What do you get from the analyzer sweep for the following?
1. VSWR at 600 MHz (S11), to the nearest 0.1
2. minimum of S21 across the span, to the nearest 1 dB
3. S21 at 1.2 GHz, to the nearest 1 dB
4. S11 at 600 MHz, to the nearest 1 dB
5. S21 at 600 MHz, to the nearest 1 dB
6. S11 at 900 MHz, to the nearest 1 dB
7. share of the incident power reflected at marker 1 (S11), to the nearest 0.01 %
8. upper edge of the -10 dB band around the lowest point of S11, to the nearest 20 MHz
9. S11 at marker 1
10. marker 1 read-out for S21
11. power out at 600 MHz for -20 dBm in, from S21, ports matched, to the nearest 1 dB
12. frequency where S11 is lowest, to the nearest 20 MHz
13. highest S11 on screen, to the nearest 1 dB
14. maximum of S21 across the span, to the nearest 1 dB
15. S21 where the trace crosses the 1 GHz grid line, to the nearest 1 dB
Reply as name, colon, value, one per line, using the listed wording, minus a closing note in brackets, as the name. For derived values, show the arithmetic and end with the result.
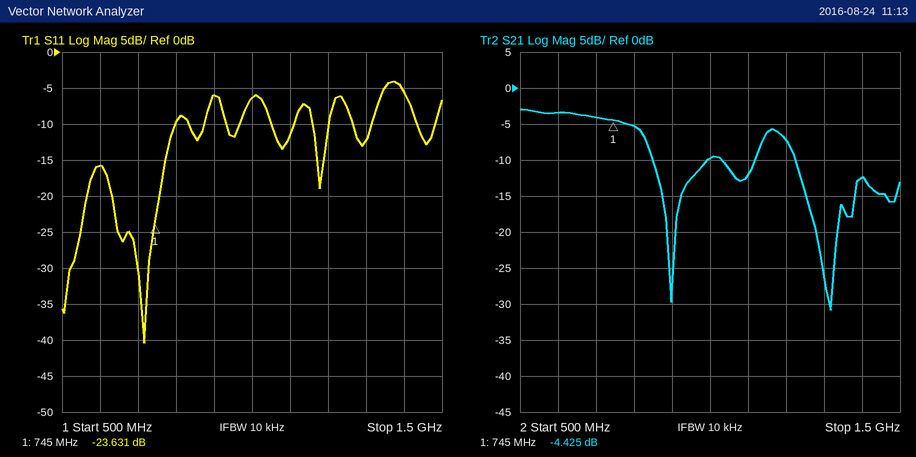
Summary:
VSWR at 600 MHz (S11), to the nearest 0.1: |Γ| = 10^(-16/20) = 0.1585; VSWR = (1 + 0.1585)/(1 − 0.1585) ≈ 1.4
minimum of S21 across the span, to the nearest 1 dB: -31 dB
S21 at 1.2 GHz, to the nearest 1 dB: -7 dB
S11 at 600 MHz, to the nearest 1 dB: -16 dB
S21 at 600 MHz, to the nearest 1 dB: -3 dB
S11 at 900 MHz, to the nearest 1 dB: -6 dB
share of the incident power reflected at marker 1 (S11), to the nearest 0.01 %: 10^(-23.631/10) ≈ 0.43 %
upper edge of the -10 dB band around the lowest point of S11, to the nearest 20 MHz: 800 MHz
S11 at marker 1: -23.631 dB
marker 1 read-out for S21: -4.425 dB
power out at 600 MHz for -20 dBm in, from S21, ports matched, to the nearest 1 dB: -20 dBm + (-3 dB) = -23 dBm
frequency where S11 is lowest, to the nearest 20 MHz: 720 MHz
highest S11 on screen, to the nearest 1 dB: -4 dB
maximum of S21 across the span, to the nearest 1 dB: -3 dB
S21 where the trace crosses the 1 GHz grid line, to the nearest 1 dB: -10 dB
